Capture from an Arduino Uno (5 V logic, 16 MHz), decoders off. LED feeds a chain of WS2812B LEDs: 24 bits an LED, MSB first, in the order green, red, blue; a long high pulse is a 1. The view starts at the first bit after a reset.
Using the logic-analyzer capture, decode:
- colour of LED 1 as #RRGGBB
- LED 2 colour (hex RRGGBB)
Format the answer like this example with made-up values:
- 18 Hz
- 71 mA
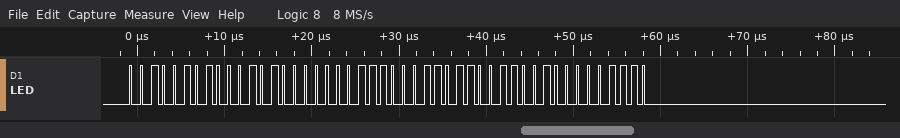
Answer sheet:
- #142507
- #321B0E
